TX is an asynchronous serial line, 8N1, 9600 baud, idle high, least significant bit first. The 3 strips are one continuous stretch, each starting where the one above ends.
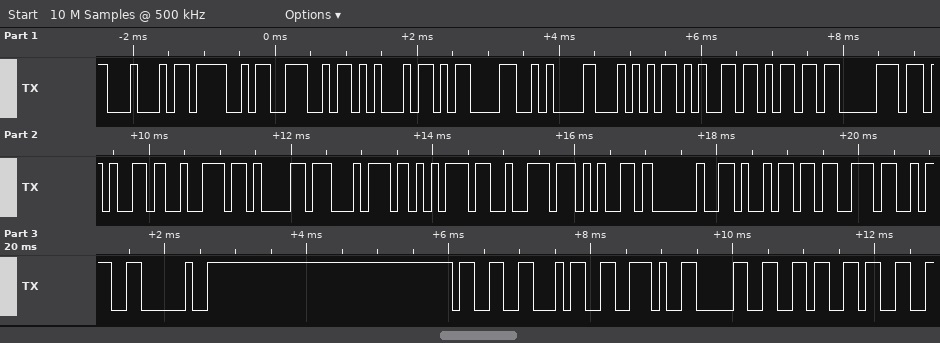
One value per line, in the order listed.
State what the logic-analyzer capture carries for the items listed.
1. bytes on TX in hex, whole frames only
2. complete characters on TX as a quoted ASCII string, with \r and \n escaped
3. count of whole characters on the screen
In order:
44 4F 4E 45 0D 0A 54 65 6D 70 65 72 61 74 75 72 65 20 69 73 3A 20 33 34 2E 30 36 33
"DONE\r\nTemperature is: 34.063"
28
